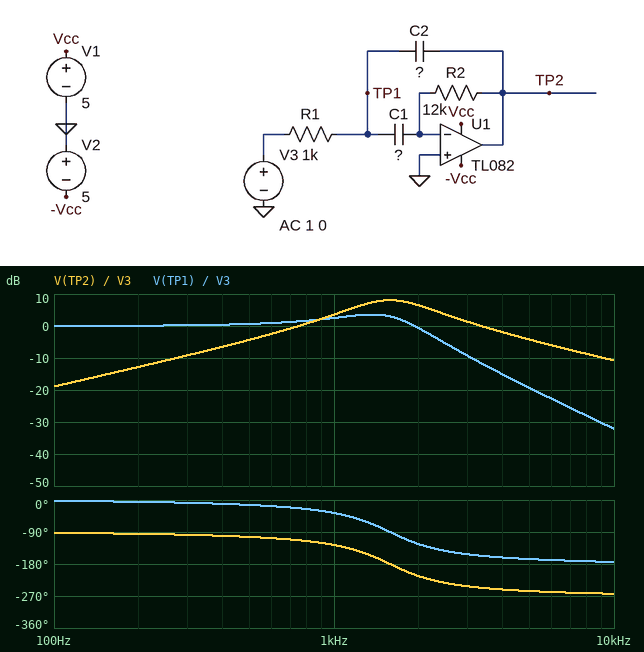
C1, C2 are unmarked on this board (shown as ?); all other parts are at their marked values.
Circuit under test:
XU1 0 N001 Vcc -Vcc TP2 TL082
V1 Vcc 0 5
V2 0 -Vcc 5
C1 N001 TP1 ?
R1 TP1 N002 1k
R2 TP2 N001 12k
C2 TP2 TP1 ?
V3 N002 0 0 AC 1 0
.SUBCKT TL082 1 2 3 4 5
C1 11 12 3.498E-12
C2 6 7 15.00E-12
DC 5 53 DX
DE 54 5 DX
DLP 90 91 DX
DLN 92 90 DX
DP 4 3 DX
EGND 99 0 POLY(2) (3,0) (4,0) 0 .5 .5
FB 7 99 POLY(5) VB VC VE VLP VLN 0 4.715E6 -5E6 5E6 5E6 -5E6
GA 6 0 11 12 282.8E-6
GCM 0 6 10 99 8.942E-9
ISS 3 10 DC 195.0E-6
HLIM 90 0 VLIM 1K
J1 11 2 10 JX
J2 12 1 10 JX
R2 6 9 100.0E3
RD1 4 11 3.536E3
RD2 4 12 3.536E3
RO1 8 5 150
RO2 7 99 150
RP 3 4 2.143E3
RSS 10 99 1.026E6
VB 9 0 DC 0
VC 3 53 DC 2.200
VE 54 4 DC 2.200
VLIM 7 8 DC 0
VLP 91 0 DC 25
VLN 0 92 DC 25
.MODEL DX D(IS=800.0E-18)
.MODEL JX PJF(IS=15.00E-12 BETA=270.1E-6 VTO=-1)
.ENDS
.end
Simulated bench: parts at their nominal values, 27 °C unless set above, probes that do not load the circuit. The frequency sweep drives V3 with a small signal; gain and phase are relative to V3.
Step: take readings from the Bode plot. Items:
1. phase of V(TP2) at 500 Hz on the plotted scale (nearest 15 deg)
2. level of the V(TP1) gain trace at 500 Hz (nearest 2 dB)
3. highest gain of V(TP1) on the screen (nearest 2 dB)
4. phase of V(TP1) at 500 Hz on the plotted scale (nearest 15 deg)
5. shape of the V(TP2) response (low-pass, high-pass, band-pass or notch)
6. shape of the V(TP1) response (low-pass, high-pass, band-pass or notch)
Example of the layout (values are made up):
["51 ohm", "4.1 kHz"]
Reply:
["-105 deg", "0 dB", "4 dB", "-15 deg", "band-pass", "low-pass"]
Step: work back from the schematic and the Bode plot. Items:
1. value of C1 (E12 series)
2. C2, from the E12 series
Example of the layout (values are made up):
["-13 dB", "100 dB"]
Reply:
["15 nF", "56 nF"]
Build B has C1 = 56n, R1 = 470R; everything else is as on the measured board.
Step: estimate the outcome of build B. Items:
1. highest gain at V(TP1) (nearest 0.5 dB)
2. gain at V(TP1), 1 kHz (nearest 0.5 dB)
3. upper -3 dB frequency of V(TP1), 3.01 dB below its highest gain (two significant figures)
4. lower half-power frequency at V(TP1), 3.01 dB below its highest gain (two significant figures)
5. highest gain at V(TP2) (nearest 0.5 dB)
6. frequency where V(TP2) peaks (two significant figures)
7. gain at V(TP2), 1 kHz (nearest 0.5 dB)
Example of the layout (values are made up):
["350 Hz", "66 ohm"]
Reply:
["8.0 dB", "7.0 dB", "1.4 kHz", "870 Hz", "22.0 dB", "1.2 kHz", "19.5 dB"]
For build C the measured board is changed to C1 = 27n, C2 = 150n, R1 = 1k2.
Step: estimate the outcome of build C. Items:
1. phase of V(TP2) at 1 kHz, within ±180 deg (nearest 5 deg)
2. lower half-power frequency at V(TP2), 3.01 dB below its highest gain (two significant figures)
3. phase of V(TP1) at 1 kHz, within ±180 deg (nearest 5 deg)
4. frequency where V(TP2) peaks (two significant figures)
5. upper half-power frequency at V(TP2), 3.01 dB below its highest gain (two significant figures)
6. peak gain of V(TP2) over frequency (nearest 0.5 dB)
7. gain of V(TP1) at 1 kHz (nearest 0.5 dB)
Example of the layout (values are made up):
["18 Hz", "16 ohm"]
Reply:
["135 deg", "430 Hz", "-135 deg", "660 Hz", "1.0 kHz", "3.5 dB", "-5.5 dB"]
